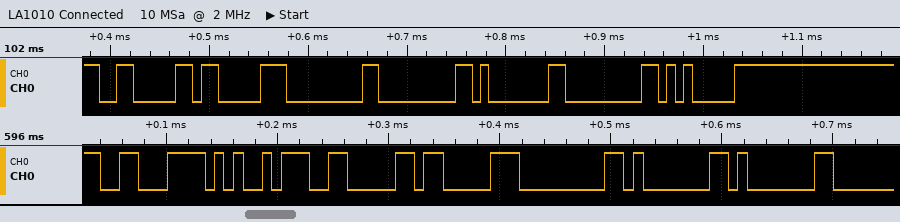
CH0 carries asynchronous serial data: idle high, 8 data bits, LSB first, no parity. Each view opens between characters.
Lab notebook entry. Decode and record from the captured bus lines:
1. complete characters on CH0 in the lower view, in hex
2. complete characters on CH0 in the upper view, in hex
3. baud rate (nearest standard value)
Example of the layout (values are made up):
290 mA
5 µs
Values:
C6, A5, 06, 83, 00, 01, 01
06, 83, 00, 00, 01, 00, 05
115200 baud
